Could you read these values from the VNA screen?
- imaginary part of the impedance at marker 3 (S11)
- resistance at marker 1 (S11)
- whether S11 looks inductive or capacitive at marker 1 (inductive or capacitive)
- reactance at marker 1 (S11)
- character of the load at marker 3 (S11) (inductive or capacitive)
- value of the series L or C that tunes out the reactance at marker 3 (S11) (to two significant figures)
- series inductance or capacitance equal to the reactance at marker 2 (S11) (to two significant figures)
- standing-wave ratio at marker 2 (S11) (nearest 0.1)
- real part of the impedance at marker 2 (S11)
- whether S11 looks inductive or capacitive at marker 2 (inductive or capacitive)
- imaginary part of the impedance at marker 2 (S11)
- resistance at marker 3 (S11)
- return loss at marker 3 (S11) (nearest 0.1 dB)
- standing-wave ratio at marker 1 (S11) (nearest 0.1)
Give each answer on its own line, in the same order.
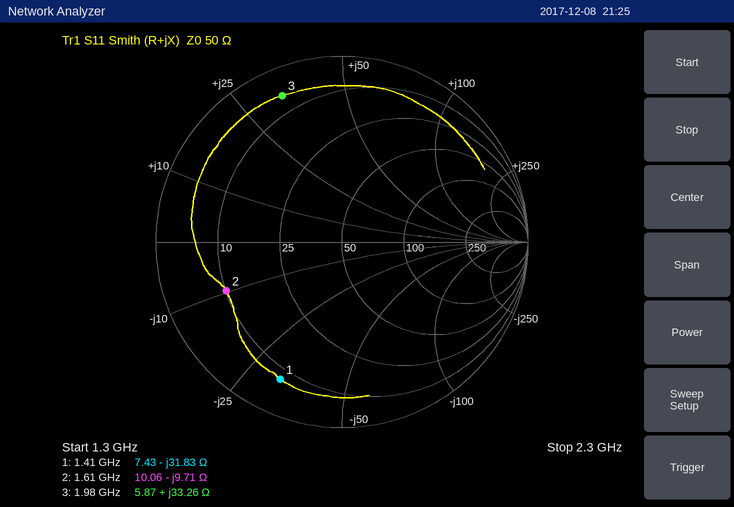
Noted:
+33.26 Ω
7.43 Ω
capacitive
-31.83 Ω
inductive
2.4 pF
10 pF
5.2
10.06 Ω
capacitive
-9.71 Ω
5.87 Ω
1.4 dB
9.5
